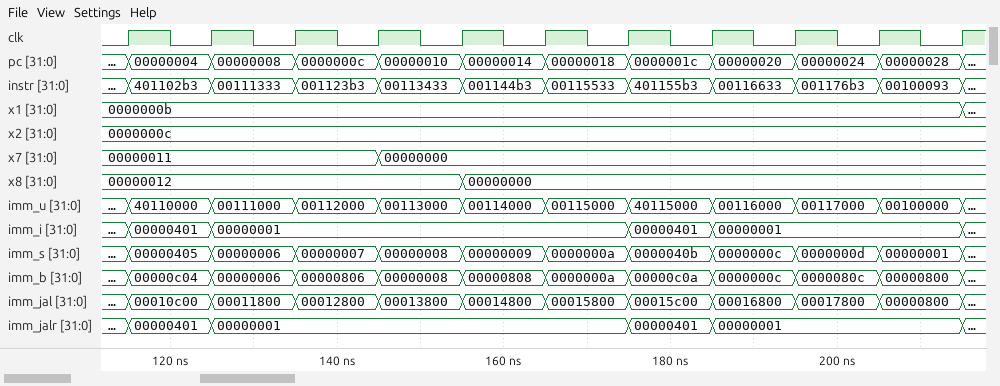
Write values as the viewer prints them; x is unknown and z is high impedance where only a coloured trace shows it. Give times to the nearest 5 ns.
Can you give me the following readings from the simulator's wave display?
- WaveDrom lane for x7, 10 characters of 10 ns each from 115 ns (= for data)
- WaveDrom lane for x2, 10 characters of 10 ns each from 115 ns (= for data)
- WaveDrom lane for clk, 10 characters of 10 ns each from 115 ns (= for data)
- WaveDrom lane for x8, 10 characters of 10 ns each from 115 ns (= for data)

{name: 'x7', wave: '=..=......', data: '00000011 00000000'}
{name: 'x2', wave: '=.........', data: '0000000c'}
{name: 'clk', wave: 'p.........'}
{name: 'x8', wave: '=...=.....', data: '00000012 00000000'}
